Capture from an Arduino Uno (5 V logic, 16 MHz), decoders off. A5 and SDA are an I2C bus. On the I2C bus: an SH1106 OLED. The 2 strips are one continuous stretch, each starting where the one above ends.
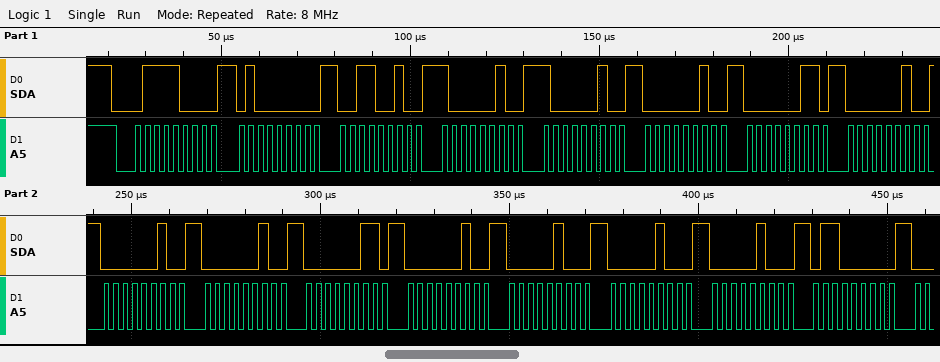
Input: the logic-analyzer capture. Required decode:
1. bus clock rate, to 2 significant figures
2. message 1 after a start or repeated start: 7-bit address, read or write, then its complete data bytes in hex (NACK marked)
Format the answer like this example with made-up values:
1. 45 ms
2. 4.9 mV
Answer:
1. 400 kHz
2. 0x3C write: 40 32 82 82 02 03 02 02 02 03 02 04 04 04 60
